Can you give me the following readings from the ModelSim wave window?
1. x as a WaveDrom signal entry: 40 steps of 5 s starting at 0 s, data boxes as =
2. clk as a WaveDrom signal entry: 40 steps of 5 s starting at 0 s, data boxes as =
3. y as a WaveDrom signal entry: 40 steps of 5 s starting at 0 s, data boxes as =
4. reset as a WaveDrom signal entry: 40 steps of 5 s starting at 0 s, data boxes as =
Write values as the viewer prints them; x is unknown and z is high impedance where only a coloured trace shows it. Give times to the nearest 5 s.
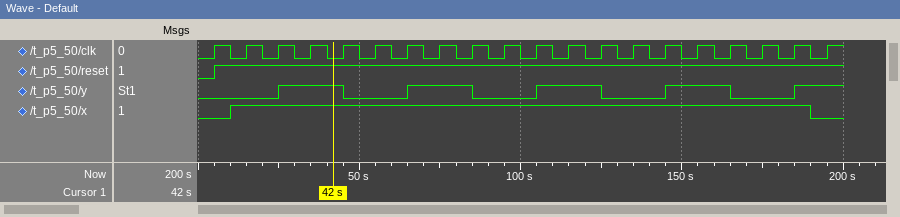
{name: 'x', wave: '0.1...................................0.'}
{name: 'clk', wave: '0101010101010101010101010101010101010101'}
{name: 'y', wave: '0....1...0...1...0...1...0...1...0...1..'}
{name: 'reset', wave: '01......................................'}
